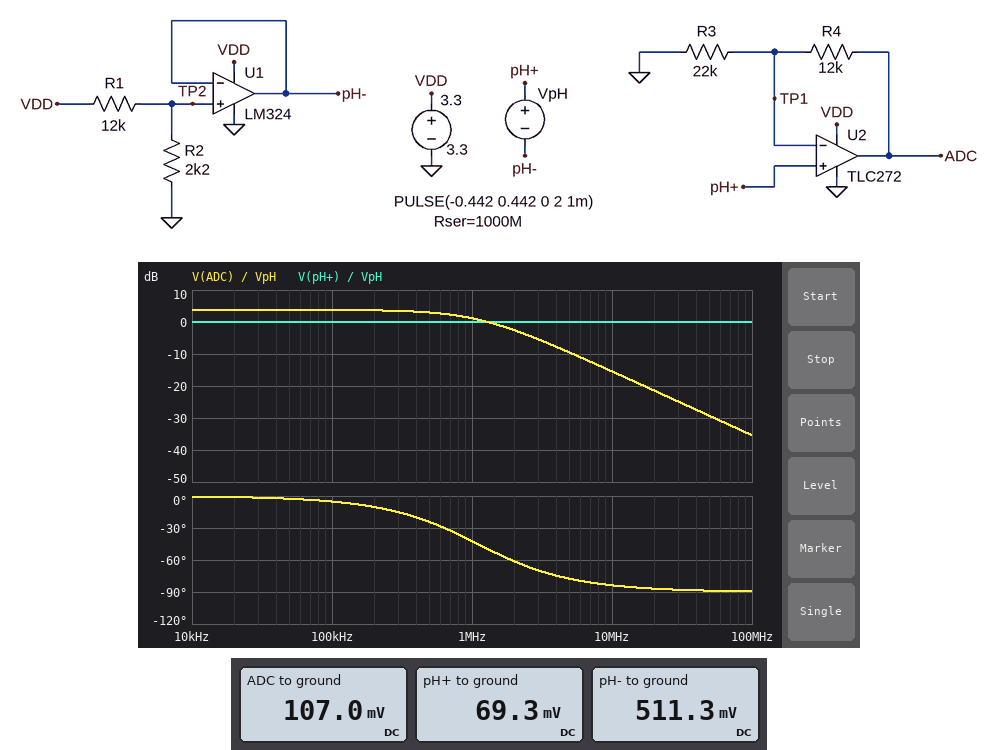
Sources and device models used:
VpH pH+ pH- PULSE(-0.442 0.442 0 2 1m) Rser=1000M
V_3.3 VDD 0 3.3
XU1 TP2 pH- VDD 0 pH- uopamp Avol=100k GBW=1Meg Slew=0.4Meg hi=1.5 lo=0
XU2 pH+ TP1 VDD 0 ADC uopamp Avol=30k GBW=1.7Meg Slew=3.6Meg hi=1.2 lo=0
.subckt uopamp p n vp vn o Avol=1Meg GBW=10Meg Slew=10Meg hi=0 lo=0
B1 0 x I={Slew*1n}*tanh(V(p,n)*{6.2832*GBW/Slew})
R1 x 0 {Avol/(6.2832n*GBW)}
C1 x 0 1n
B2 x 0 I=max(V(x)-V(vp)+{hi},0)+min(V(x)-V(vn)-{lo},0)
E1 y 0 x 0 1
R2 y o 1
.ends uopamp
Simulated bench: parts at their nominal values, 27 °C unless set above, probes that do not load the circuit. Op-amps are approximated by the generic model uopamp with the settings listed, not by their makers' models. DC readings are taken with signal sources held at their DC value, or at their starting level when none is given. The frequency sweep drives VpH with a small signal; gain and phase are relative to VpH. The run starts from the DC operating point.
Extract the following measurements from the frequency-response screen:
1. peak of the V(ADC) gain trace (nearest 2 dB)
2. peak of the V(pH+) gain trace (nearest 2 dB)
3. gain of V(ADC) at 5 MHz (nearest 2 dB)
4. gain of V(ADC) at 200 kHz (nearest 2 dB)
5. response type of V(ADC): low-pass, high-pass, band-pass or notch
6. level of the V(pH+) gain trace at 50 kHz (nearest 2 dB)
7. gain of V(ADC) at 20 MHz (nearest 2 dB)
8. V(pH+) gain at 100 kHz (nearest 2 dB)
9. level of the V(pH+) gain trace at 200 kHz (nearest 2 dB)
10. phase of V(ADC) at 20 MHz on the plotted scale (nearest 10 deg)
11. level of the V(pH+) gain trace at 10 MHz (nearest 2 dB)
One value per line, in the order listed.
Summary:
4 dB
0 dB
-10 dB
4 dB
low-pass
0 dB
-22 dB
0 dB
0 dB
-90 deg
0 dB
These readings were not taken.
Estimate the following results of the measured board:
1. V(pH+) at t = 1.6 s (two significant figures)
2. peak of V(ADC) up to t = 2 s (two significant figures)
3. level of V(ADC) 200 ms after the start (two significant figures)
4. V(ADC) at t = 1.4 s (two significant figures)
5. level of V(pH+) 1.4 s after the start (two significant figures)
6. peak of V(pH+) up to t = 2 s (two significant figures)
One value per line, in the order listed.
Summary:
780 mV
1.5 V
240 mV
1.1 V
690 mV
950 mV
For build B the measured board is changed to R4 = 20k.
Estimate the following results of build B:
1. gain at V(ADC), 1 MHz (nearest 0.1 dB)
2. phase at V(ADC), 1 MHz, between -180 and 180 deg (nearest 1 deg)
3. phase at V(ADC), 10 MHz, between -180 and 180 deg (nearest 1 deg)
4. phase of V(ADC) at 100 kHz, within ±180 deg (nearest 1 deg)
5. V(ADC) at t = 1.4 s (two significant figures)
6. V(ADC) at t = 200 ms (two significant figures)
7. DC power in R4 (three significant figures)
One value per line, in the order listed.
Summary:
2.1 dB
-48 deg
-85 deg
-6 deg
1.3 V
300 mV
198 nW
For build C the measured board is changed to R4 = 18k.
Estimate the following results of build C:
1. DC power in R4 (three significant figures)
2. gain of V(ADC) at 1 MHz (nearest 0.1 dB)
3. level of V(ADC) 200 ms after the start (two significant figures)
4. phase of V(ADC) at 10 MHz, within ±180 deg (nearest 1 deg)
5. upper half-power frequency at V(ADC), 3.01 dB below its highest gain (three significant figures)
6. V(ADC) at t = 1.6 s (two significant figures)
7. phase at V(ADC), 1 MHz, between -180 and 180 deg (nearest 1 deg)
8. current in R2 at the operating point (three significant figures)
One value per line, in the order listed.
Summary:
178 nW
1.9 dB
290 mV
-85 deg
935 kHz
1.4 V
-47 deg
232 µA
